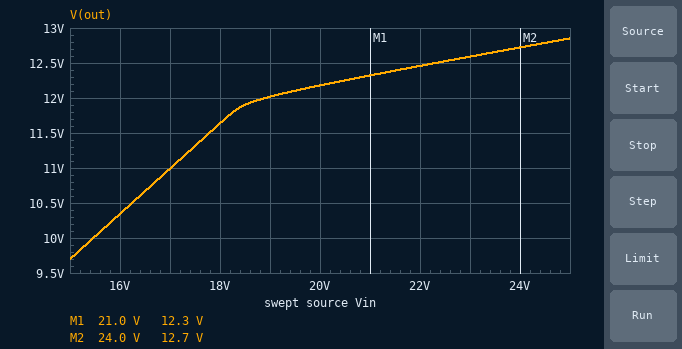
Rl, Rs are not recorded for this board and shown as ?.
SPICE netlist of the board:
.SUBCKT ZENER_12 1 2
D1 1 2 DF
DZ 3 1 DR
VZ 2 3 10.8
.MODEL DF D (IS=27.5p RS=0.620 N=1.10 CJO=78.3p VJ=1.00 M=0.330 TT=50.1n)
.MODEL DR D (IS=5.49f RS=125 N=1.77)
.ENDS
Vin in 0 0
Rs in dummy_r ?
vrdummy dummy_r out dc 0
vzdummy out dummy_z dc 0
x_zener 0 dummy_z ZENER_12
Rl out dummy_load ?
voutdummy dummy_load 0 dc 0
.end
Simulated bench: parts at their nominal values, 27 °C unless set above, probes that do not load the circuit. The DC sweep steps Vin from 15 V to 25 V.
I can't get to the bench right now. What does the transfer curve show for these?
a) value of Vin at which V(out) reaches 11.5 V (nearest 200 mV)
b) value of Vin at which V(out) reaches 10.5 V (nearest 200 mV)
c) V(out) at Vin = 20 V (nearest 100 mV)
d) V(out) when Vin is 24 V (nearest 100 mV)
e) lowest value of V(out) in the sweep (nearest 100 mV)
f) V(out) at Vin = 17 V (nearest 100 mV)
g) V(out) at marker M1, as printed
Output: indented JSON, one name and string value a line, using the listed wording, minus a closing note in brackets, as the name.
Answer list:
{
  "value of Vin at which V(out) reaches 11.5 V": "17.8 V",
  "value of Vin at which V(out) reaches 10.5 V": "16.2 V",
  "V(out) at Vin = 20 V": "12.2 V",
  "V(out) when Vin is 24 V": "12.7 V",
  "lowest value of V(out) in the sweep": "9.7 V",
  "V(out) at Vin = 17 V": "11.0 V",
  "V(out) at marker M1, as printed": "12.3 V"
}
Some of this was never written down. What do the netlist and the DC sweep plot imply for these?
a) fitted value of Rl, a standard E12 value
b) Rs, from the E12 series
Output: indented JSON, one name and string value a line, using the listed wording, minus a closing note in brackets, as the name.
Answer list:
{
  "fitted value of Rl, a standard E12 value": "1.5 kΩ",
  "Rs, from the E12 series": "820 Ω"
}
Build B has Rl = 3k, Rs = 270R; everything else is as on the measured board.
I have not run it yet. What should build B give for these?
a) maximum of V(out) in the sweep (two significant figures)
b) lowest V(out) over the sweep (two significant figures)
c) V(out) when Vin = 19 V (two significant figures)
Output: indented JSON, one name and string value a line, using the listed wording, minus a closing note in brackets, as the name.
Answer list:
{
  "maximum of V(out) in the sweep": "16 V",
  "lowest V(out) over the sweep": "13 V",
  "V(out) when Vin = 19 V": "14 V"
}
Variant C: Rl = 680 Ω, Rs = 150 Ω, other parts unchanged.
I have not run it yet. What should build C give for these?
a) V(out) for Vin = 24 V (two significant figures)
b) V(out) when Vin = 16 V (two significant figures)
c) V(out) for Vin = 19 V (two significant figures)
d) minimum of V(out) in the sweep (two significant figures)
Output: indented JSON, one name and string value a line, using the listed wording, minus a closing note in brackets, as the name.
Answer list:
{
  "V(out) for Vin = 24 V": "16 V",
  "V(out) when Vin = 16 V": "13 V",
  "V(out) for Vin = 19 V": "14 V",
  "minimum of V(out) in the sweep": "12 V"
}
